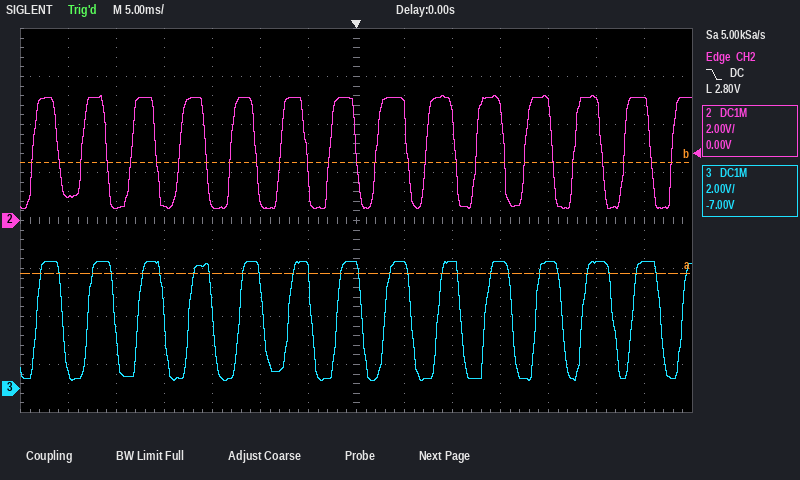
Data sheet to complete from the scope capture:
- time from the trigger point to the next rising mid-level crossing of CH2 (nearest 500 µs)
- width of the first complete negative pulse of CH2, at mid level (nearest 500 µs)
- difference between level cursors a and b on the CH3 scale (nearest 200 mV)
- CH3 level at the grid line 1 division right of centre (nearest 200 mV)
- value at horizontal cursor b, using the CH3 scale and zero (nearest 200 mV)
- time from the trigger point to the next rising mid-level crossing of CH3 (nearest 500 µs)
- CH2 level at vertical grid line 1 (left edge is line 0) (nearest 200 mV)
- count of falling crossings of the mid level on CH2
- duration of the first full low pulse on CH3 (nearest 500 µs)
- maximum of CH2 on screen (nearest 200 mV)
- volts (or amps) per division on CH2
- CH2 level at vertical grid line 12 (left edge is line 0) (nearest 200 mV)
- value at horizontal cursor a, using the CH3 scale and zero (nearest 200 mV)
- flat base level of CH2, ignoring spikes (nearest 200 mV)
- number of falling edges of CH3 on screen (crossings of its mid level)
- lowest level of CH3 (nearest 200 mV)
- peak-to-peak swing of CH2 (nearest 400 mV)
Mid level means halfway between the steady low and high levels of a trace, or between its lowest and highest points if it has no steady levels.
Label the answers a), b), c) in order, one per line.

a) 2.0 ms
b) 2.5 ms
c) 4.6 V
d) 5.2 V
e) 9.4 V
f) 3.0 ms
g) 1.0 V
h) 13
i) 2.5 ms
j) 5.2 V
k) 2 V
l) 5.0 V
m) 4.8 V
n) 600 mV
o) 13
p) 400 mV
q) 4.8 V
